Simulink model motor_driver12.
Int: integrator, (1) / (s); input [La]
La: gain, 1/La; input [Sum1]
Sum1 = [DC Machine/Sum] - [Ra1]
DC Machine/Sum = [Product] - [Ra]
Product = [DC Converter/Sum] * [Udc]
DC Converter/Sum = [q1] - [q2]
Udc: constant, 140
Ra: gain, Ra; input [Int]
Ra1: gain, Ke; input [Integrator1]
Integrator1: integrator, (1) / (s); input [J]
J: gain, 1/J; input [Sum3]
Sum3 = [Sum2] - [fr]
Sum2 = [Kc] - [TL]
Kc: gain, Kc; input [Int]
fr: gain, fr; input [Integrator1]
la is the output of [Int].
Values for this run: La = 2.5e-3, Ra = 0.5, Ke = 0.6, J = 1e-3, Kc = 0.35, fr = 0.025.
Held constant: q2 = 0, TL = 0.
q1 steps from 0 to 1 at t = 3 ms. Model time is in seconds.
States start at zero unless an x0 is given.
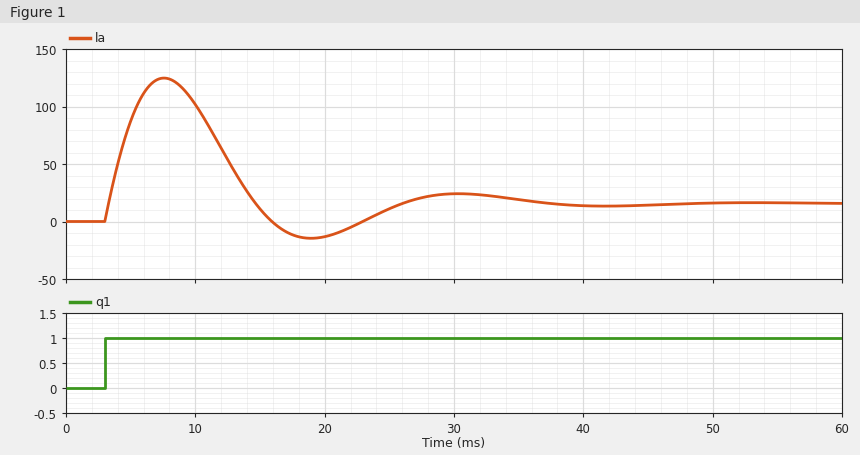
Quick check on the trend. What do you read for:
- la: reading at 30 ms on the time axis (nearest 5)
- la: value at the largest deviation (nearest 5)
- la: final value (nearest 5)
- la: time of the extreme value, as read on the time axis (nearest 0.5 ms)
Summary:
25
125
15
7.5 ms
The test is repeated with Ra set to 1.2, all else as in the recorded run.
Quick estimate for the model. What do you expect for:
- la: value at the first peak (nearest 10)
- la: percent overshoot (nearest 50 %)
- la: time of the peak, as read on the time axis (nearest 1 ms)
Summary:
80
450 %
7 ms
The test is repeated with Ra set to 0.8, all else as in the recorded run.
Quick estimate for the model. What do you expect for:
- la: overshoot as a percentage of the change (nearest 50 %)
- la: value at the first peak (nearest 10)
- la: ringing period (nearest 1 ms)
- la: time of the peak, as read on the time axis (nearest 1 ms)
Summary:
550 %
100
25 ms
7 ms
